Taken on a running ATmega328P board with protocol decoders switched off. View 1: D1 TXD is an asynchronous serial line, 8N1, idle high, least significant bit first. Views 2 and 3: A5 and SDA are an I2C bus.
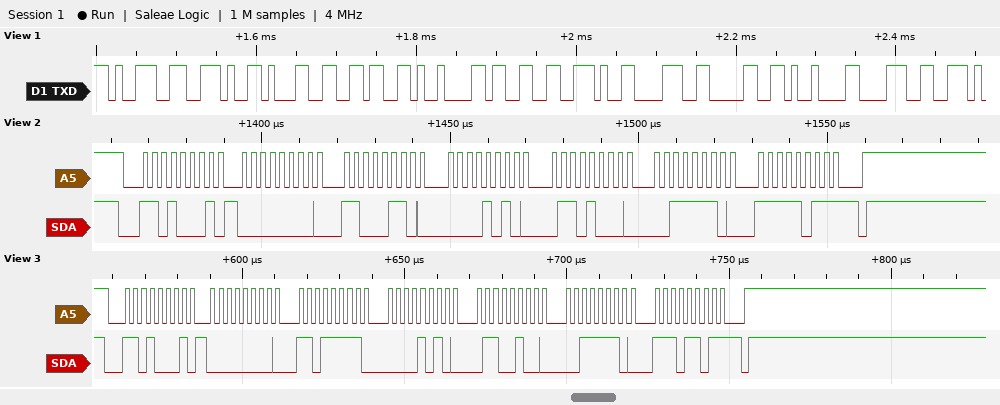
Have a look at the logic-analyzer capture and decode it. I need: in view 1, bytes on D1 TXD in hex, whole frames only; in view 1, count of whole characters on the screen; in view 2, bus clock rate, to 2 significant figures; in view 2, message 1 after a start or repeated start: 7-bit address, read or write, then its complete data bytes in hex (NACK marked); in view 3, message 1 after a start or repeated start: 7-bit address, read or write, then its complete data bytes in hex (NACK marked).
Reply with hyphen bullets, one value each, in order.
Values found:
- 39 2E 31 36 09 33 2E 38 30 09 38
- 11
- 400 kHz
- 0x68 read: 00 C6 0A 68 3E FB NACK
- 0x68 read: 00 DF 0A 64 3E ED NACK
